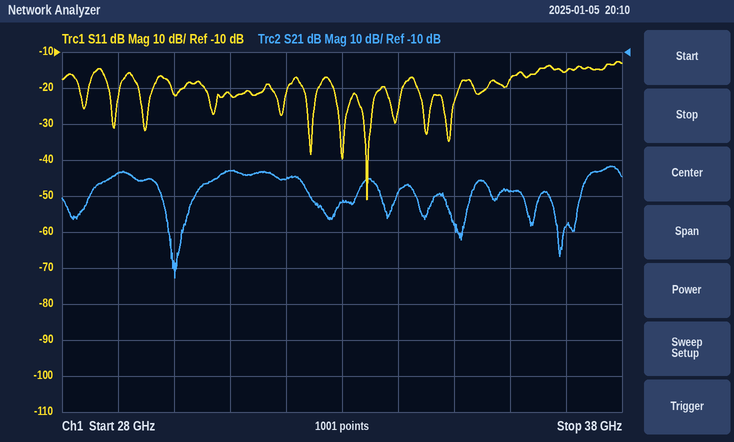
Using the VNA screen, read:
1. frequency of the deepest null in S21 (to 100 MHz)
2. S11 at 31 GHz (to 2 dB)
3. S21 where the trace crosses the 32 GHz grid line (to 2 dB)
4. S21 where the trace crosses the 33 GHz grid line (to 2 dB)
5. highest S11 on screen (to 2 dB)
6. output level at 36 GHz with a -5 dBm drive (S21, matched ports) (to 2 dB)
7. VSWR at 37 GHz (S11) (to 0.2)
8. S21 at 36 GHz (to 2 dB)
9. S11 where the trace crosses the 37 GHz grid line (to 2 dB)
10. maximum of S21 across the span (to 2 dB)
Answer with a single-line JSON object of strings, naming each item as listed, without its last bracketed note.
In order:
{"frequency of the deepest null in S21": "30.0 GHz", "S11 at 31 GHz": "-22 dB", "S21 where the trace crosses the 32 GHz grid line": "-46 dB", "S21 where the trace crosses the 33 GHz grid line": "-52 dB", "highest S11 on screen": "-12 dB", "output level at 36 GHz with a -5 dBm drive (S21, matched ports)": "-54 dBm", "VSWR at 37 GHz (S11)": "1.4", "S21 at 36 GHz": "-48 dB", "S11 where the trace crosses the 37 GHz grid line": "-16 dB", "maximum of S21 across the span": "-42 dB"}
